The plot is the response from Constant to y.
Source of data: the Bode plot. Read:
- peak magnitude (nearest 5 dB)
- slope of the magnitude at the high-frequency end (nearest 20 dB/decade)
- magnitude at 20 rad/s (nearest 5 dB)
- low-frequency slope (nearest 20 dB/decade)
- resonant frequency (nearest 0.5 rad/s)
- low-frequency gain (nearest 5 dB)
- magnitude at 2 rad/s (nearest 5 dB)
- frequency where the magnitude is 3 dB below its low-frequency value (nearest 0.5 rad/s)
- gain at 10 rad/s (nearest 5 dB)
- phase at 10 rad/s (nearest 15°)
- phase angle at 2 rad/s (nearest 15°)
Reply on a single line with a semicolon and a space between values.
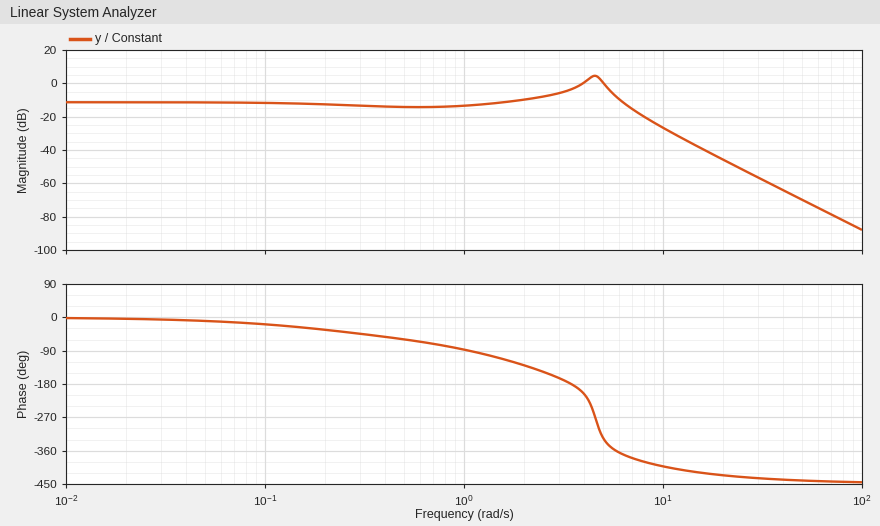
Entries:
5 dB; -60 dB/decade; -45 dB; 0 dB/decade; 4.5 rad/s; -10 dB; -10 dB; 7.0 rad/s; -25 dB; -405°; -135°
